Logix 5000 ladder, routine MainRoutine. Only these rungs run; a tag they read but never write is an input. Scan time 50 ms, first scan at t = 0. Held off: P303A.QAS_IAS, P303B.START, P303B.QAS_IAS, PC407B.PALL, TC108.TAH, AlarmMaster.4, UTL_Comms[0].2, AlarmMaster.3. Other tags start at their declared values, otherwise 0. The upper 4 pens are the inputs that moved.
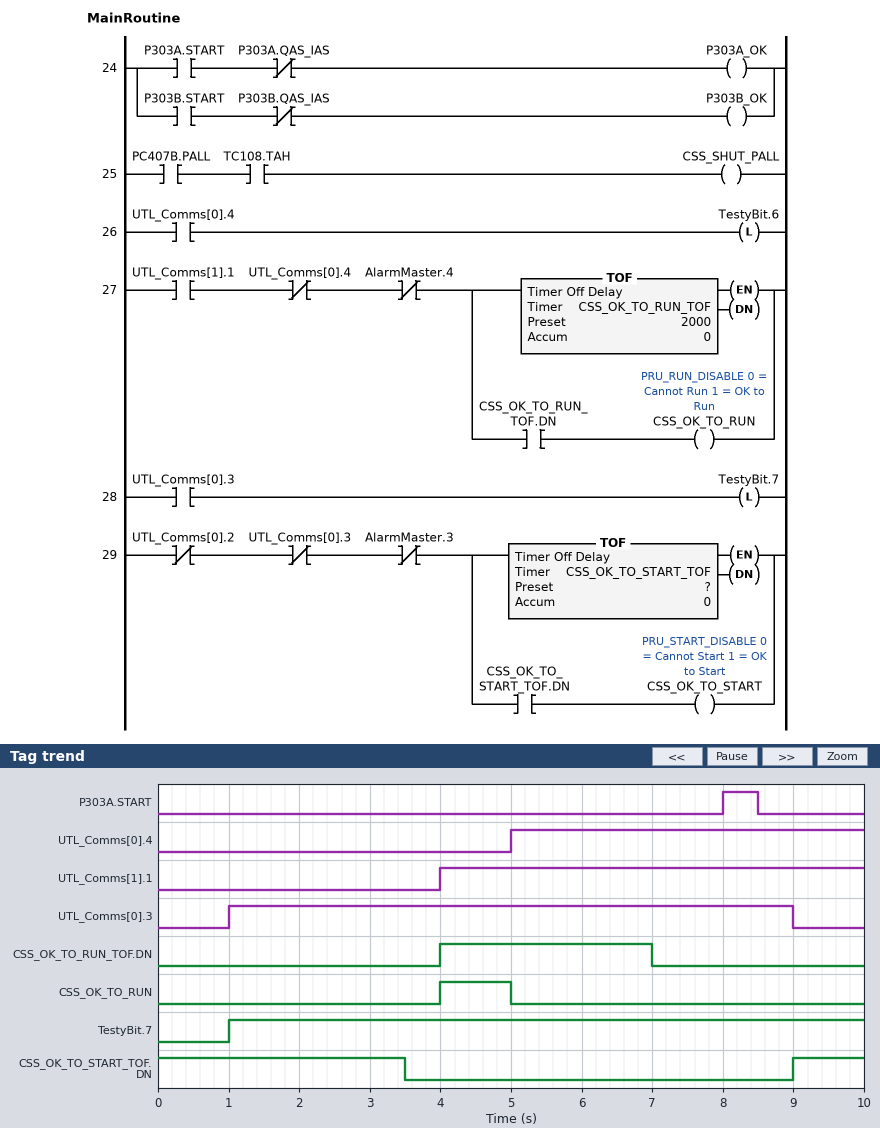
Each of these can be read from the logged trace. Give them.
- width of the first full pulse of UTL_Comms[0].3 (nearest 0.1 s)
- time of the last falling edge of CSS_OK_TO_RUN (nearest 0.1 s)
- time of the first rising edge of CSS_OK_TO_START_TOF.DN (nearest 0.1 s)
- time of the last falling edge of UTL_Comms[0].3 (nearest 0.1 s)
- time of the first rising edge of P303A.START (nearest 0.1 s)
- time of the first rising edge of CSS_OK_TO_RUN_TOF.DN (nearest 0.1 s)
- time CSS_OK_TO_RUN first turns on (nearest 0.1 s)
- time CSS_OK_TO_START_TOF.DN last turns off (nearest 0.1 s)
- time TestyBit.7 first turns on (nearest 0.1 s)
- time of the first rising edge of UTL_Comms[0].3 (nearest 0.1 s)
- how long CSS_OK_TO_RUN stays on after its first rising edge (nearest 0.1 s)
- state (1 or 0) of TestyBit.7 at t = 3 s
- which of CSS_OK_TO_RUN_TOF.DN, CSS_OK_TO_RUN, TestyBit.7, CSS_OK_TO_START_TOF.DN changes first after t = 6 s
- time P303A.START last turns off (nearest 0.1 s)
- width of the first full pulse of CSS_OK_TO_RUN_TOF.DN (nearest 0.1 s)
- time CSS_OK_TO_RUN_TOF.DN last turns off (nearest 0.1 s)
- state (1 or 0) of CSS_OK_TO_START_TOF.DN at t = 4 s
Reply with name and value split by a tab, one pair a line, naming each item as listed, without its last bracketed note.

width of the first full pulse of UTL_Comms[0].3	8.0 s
time of the last falling edge of CSS_OK_TO_RUN	5.0 s
time of the first rising edge of CSS_OK_TO_START_TOF.DN	9.0 s
time of the last falling edge of UTL_Comms[0].3	9.0 s
time of the first rising edge of P303A.START	8.0 s
time of the first rising edge of CSS_OK_TO_RUN_TOF.DN	4.0 s
time CSS_OK_TO_RUN first turns on	4.0 s
time CSS_OK_TO_START_TOF.DN last turns off	3.5 s
time TestyBit.7 first turns on	1.0 s
time of the first rising edge of UTL_Comms[0].3	1.0 s
how long CSS_OK_TO_RUN stays on after its first rising edge	1.0 s
state (1 or 0) of TestyBit.7 at t = 3 s	1
which of CSS_OK_TO_RUN_TOF.DN, CSS_OK_TO_RUN, TestyBit.7, CSS_OK_TO_START_TOF.DN changes first after t = 6 s	CSS_OK_TO_RUN_TOF.DN
time P303A.START last turns off	8.5 s
width of the first full pulse of CSS_OK_TO_RUN_TOF.DN	3.0 s
time CSS_OK_TO_RUN_TOF.DN last turns off	7.0 s
state (1 or 0) of CSS_OK_TO_START_TOF.DN at t = 4 s	0
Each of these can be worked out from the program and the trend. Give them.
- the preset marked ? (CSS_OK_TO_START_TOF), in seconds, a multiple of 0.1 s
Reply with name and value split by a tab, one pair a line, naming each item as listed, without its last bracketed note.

the preset marked ? (CSS_OK_TO_START_TOF), in seconds, a multiple of 0.1 s	2.5 s
